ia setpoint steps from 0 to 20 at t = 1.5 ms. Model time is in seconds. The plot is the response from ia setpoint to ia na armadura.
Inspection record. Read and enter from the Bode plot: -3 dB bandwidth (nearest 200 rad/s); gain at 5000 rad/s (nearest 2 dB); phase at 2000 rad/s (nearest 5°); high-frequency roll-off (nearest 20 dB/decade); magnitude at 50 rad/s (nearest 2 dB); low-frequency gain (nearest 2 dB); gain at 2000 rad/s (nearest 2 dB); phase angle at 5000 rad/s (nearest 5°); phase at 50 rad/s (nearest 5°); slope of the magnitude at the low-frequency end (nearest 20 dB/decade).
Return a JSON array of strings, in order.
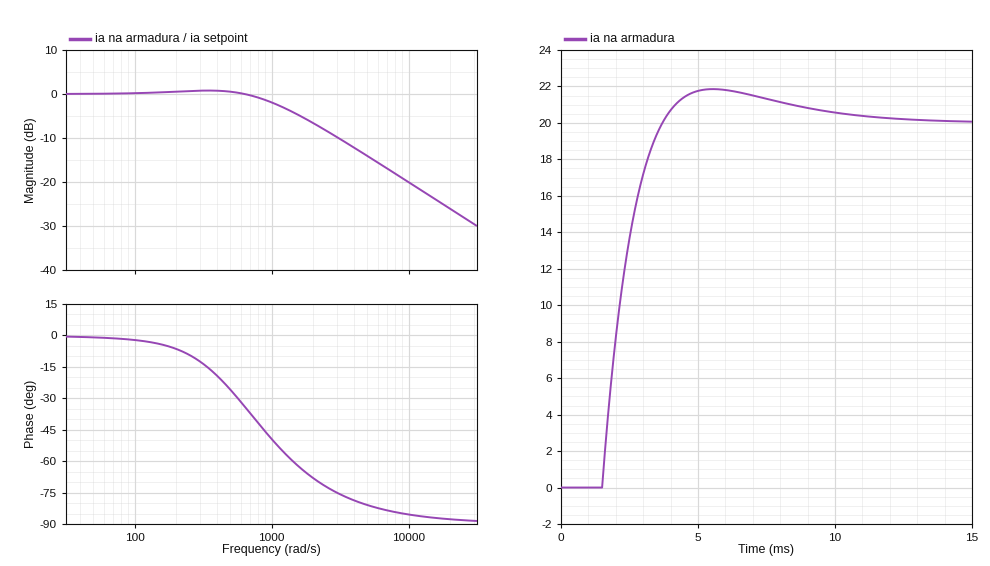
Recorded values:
["1200 rad/s", "-14 dB", "-70°", "-20 dB/decade", "0 dB", "0 dB", "-6 dB", "-80°", "0°", "0 dB/decade"]
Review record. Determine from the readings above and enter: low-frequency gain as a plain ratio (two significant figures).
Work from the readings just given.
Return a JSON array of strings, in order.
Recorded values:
["1.0"]
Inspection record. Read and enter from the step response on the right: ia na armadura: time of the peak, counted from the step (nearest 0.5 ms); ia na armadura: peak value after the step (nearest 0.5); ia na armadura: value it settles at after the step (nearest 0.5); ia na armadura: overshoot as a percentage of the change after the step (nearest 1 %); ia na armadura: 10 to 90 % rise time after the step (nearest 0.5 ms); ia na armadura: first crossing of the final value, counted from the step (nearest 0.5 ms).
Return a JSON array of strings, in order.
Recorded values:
["4.0 ms", "22.0", "20.0", "9 %", "1.5 ms", "2.0 ms"]
